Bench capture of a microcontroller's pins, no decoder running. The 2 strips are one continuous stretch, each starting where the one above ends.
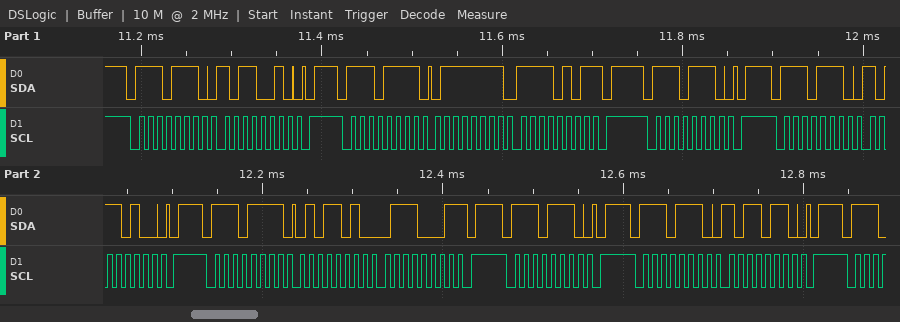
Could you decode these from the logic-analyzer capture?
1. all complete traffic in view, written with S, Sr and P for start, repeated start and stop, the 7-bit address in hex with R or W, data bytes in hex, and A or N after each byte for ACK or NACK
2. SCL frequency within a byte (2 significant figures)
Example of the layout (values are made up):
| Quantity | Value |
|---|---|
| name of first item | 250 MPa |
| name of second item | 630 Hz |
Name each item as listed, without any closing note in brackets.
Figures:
| Quantity | Value |
|---|---|
| all complete traffic in view, written with S, Sr and P for start, repeated start and stop, the 7-bit address in hex with R or W, data bytes in hex, and A or N after each byte for ACK or NACK | S 77W A B2 A P S 77R A 7F A F5 N P S 77W A P S 77W A B4 A P S 77R A 5A A 71 N P S 77W A P S 77W A B6 A P |
| SCL frequency within a byte | 100 kHz |
